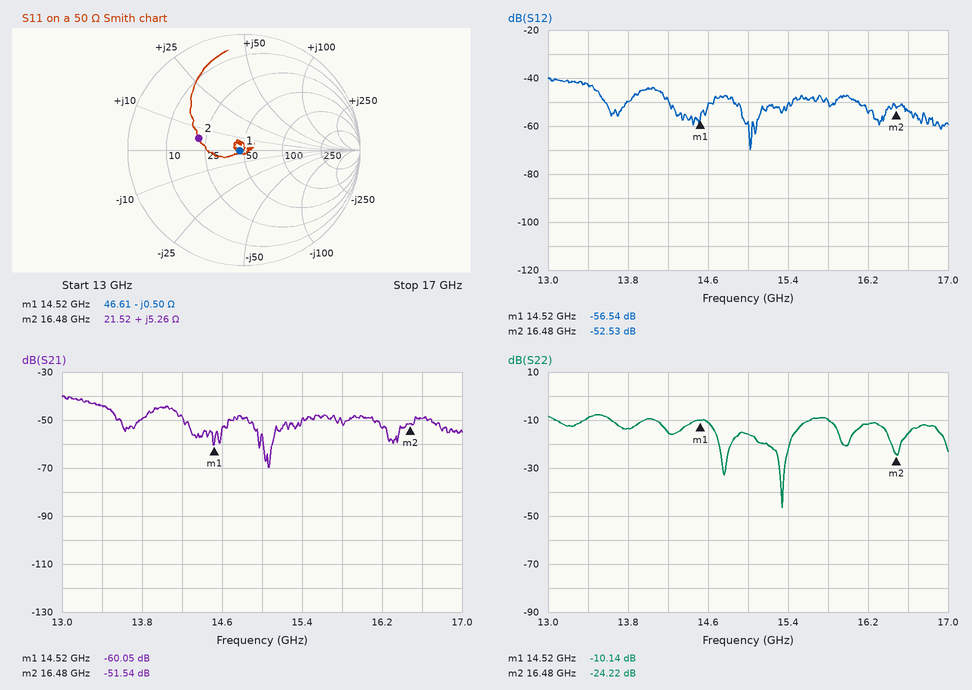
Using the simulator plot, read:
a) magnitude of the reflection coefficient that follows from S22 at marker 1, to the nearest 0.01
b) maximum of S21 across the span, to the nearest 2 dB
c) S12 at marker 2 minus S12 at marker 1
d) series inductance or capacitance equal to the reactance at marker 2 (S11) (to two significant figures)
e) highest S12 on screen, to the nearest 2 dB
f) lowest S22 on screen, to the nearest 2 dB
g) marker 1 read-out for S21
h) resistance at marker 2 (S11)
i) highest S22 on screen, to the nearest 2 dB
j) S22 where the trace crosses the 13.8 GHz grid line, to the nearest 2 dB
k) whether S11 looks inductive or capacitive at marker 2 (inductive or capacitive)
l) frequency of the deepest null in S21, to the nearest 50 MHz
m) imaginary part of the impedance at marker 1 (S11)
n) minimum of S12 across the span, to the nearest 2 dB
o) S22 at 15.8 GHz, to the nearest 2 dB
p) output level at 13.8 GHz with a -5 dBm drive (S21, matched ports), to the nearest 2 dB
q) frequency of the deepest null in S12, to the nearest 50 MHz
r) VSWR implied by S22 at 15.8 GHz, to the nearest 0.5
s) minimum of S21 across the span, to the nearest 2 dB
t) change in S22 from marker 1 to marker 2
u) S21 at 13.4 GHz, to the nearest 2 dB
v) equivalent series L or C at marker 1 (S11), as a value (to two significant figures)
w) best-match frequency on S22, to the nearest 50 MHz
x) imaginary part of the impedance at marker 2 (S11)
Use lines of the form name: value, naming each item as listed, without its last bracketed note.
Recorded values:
magnitude of the reflection coefficient that follows from S22 at marker 1, to the nearest 0.01: 0.31
maximum of S21 across the span, to the nearest 2 dB: -40 dB
S12 at marker 2 minus S12 at marker 1: 4.01 dB
series inductance or capacitance equal to the reactance at marker 2 (S11): 51 pH
highest S12 on screen, to the nearest 2 dB: -40 dB
lowest S22 on screen, to the nearest 2 dB: -46 dB
marker 1 read-out for S21: -60.05 dB
resistance at marker 2: 21.52 Ω
highest S22 on screen, to the nearest 2 dB: -8 dB
S22 where the trace crosses the 13.8 GHz grid line, to the nearest 2 dB: -14 dB
whether S11 looks inductive or capacitive at marker 2: inductive
frequency of the deepest null in S21, to the nearest 50 MHz: 15.05 GHz
imaginary part of the impedance at marker 1: -0.50 Ω
minimum of S12 across the span, to the nearest 2 dB: -70 dB
S22 at 15.8 GHz, to the nearest 2 dB: -10 dB
output level at 13.8 GHz with a -5 dBm drive (S21, matched ports), to the nearest 2 dB: -54 dBm
frequency of the deepest null in S12, to the nearest 50 MHz: 15.00 GHz
VSWR implied by S22 at 15.8 GHz, to the nearest 0.5: 2.0
minimum of S21 across the span, to the nearest 2 dB: -70 dB
change in S22 from marker 1 to marker 2: -14.08 dB
S21 at 13.4 GHz, to the nearest 2 dB: -44 dB
equivalent series L or C at marker 1 (S11), as a value: 22 pF
best-match frequency on S22, to the nearest 50 MHz: 15.35 GHz
imaginary part of the impedance at marker 2: +5.26 Ω
